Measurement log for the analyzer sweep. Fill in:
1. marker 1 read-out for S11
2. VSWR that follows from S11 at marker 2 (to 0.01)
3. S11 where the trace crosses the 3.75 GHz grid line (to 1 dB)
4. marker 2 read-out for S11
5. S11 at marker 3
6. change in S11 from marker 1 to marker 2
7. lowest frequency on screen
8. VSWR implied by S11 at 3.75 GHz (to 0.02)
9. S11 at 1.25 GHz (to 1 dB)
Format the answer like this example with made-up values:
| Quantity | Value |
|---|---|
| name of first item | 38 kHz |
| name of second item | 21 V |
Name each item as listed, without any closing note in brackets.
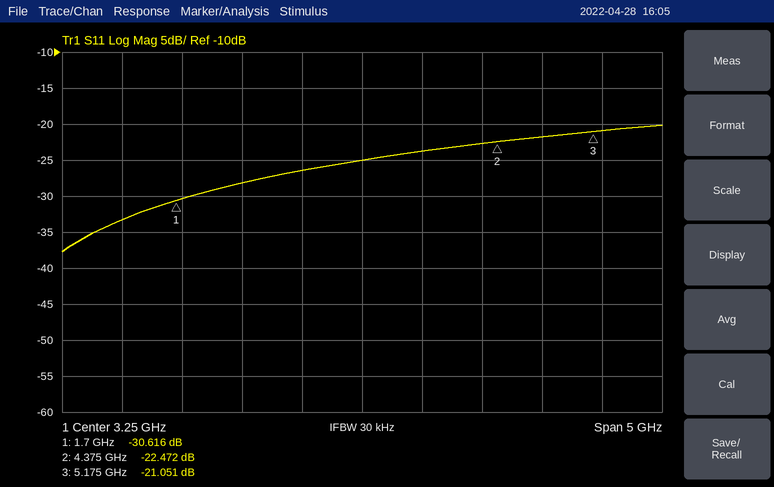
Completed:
| Quantity | Value |
|---|---|
| marker 1 read-out for S11 | -30.616 dB |
| VSWR that follows from S11 at marker 2 | 1.16 |
| S11 where the trace crosses the 3.75 GHz grid line | -24 dB |
| marker 2 read-out for S11 | -22.472 dB |
| S11 at marker 3 | -21.051 dB |
| change in S11 from marker 1 to marker 2 | 8.144 dB |
| lowest frequency on screen | 750 MHz |
| VSWR implied by S11 at 3.75 GHz | 1.14 |
| S11 at 1.25 GHz | -33 dB |
